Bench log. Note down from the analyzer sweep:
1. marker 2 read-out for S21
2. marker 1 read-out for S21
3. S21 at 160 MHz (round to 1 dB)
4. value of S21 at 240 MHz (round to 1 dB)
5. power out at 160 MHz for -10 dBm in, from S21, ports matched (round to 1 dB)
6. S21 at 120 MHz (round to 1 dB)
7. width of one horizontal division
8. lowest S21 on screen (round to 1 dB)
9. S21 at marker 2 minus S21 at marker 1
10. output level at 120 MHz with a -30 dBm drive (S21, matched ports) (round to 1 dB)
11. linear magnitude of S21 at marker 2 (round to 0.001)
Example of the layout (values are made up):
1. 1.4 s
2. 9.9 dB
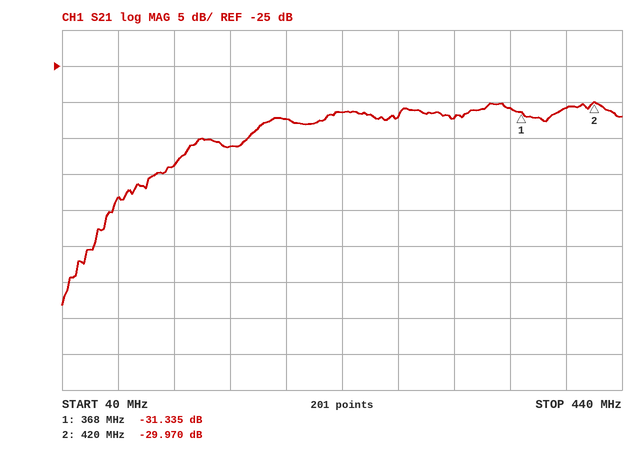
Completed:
1. -29.970 dB
2. -31.335 dB
3. -36 dB
4. -31 dB
5. -46 dBm
6. -39 dB
7. 40 MHz
8. -58 dB
9. 1.365 dB
10. -69 dBm
11. 0.032
